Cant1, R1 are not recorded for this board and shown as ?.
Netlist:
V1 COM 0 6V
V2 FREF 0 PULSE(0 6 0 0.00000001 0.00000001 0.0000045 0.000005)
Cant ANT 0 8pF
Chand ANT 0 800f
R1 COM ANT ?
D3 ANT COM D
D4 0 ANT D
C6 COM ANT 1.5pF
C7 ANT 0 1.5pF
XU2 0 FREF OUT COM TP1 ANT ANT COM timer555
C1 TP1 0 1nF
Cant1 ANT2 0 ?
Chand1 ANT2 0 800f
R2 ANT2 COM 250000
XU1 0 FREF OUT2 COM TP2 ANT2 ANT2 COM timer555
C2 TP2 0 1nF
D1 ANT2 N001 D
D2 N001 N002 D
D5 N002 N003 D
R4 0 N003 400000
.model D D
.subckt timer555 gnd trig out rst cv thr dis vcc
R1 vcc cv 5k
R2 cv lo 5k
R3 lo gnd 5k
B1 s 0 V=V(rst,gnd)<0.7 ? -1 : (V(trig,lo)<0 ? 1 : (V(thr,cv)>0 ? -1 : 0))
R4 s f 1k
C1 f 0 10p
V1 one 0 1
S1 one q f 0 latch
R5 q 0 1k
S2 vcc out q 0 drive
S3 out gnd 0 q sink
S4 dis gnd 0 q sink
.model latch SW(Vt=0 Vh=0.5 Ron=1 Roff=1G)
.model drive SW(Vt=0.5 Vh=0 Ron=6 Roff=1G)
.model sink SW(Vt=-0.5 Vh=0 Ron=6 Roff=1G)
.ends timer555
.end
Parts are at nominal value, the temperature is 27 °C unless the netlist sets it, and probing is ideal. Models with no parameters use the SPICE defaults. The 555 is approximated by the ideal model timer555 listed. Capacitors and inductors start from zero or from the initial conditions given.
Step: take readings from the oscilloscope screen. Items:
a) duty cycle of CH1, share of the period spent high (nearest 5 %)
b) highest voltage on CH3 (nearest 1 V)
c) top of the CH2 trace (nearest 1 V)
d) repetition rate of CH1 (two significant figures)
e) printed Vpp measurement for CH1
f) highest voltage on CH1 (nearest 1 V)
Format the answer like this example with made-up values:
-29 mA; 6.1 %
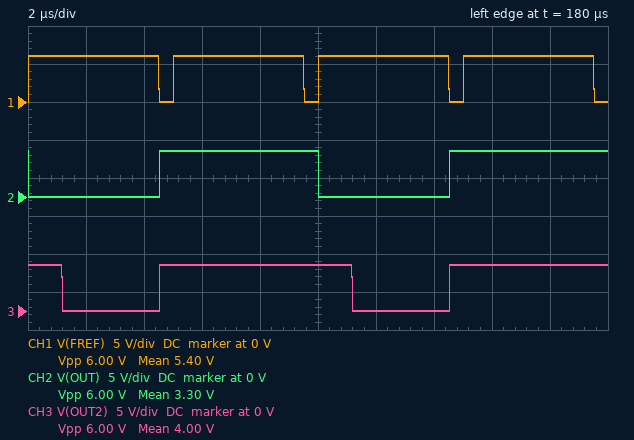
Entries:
90 %; 6 V; 6 V; 200 kHz; 6.00 V; 6 V
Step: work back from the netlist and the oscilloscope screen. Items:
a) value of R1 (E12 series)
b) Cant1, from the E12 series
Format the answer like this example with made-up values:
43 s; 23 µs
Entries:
390 kΩ; 15 pF
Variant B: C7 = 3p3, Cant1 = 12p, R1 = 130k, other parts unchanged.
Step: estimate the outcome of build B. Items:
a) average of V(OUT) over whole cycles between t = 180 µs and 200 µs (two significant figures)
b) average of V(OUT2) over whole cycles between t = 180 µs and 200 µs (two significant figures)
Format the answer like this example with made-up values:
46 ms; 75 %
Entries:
2.3 V; 3.3 V
